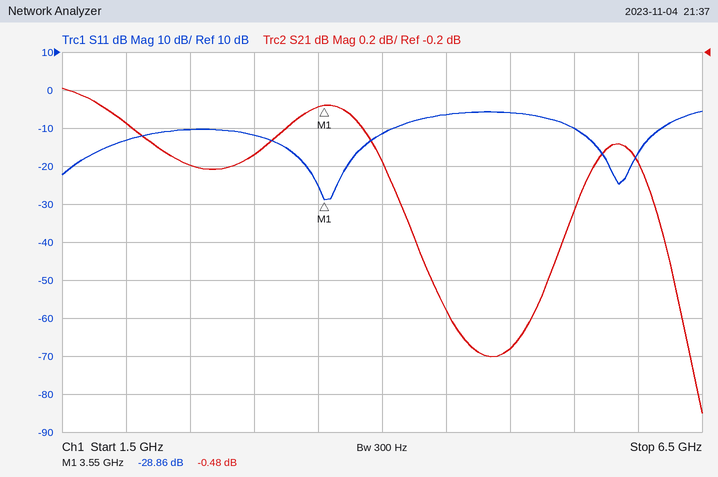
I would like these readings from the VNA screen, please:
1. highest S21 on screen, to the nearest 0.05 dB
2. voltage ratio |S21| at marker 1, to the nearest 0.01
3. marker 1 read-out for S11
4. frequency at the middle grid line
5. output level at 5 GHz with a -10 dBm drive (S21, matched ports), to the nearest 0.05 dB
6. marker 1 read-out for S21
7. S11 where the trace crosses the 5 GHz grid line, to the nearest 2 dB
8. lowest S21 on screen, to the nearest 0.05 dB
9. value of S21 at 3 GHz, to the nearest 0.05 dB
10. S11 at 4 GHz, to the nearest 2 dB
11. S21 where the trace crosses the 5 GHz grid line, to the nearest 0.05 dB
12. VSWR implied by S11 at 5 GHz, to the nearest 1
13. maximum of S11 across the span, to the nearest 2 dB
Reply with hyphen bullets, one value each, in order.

- -0.40 dB
- 0.95
- -28.86 dB
- 4 GHz
- -11.75 dBm
- -0.48 dB
- -6 dB
- -2.10 dB
- -0.75 dB
- -12 dB
- -1.75 dB
- 3
- -6 dB
